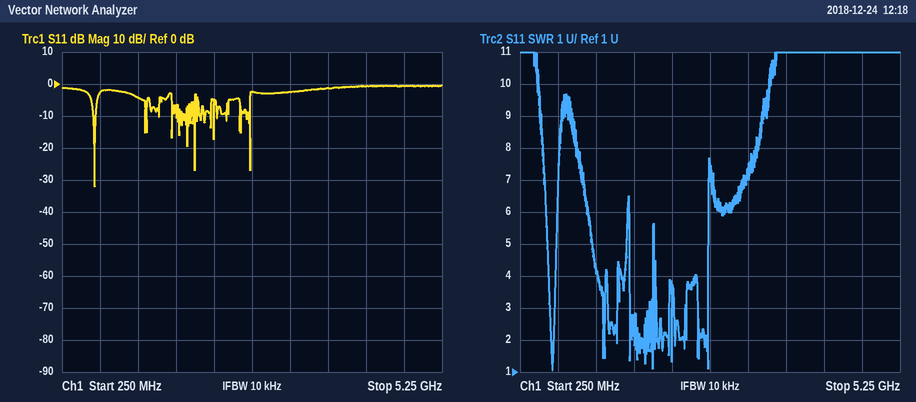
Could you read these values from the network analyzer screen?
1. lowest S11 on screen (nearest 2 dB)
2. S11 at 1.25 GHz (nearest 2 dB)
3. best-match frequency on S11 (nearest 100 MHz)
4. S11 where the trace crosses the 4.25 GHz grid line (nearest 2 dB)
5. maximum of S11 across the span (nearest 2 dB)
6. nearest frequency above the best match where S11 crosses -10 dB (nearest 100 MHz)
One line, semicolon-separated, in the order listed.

-32 dB; -4 dB; 700 MHz; 0 dB; 0 dB; 700 MHz
